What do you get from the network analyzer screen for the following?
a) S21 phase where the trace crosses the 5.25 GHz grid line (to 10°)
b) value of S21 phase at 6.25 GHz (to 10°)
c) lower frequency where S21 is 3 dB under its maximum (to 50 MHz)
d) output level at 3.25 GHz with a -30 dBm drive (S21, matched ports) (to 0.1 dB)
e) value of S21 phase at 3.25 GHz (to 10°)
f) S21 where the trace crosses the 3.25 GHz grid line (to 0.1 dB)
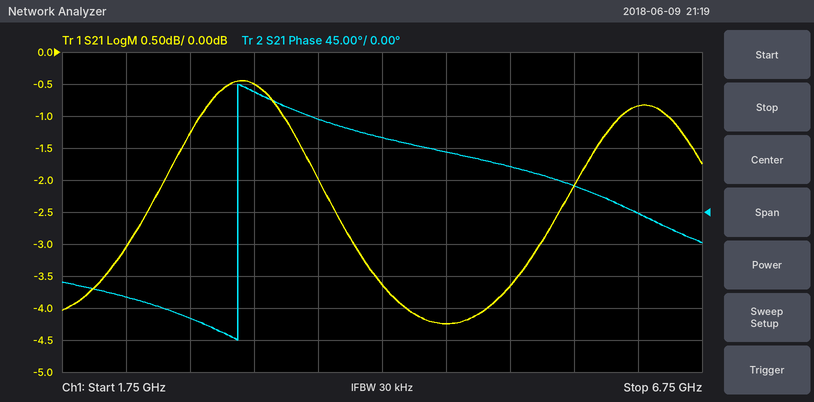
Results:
60°
0°
2.10 GHz
-30.5 dBm
170°
-0.5 dB
